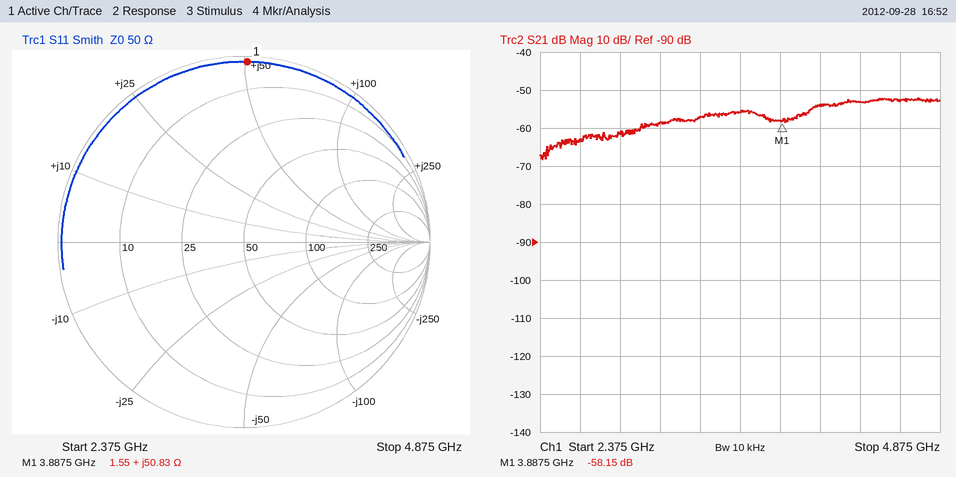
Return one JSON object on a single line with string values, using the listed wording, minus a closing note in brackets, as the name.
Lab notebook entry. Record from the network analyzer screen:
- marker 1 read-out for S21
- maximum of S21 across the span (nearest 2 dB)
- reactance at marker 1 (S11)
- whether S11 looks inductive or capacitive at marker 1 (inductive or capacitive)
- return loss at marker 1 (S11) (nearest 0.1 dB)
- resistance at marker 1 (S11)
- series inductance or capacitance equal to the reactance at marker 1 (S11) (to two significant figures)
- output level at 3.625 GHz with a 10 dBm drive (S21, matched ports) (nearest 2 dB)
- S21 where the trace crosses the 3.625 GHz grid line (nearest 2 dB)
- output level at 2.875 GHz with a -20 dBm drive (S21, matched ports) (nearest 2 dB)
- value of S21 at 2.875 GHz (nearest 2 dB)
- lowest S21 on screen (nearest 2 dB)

{"marker 1 read-out for S21": "-58.15 dB", "maximum of S21 across the span": "-52 dB", "reactance at marker 1": "+50.83 Ω", "whether S11 looks inductive or capacitive at marker 1": "inductive", "return loss at marker 1 (S11)": "0.3 dB", "resistance at marker 1": "1.55 Ω", "series inductance or capacitance equal to the reactance at marker 1 (S11)": "2.1 nH", "output level at 3.625 GHz with a 10 dBm drive (S21, matched ports)": "-46 dBm", "S21 where the trace crosses the 3.625 GHz grid line": "-56 dB", "output level at 2.875 GHz with a -20 dBm drive (S21, matched ports)": "-82 dBm", "value of S21 at 2.875 GHz": "-62 dB", "lowest S21 on screen": "-68 dB"}
